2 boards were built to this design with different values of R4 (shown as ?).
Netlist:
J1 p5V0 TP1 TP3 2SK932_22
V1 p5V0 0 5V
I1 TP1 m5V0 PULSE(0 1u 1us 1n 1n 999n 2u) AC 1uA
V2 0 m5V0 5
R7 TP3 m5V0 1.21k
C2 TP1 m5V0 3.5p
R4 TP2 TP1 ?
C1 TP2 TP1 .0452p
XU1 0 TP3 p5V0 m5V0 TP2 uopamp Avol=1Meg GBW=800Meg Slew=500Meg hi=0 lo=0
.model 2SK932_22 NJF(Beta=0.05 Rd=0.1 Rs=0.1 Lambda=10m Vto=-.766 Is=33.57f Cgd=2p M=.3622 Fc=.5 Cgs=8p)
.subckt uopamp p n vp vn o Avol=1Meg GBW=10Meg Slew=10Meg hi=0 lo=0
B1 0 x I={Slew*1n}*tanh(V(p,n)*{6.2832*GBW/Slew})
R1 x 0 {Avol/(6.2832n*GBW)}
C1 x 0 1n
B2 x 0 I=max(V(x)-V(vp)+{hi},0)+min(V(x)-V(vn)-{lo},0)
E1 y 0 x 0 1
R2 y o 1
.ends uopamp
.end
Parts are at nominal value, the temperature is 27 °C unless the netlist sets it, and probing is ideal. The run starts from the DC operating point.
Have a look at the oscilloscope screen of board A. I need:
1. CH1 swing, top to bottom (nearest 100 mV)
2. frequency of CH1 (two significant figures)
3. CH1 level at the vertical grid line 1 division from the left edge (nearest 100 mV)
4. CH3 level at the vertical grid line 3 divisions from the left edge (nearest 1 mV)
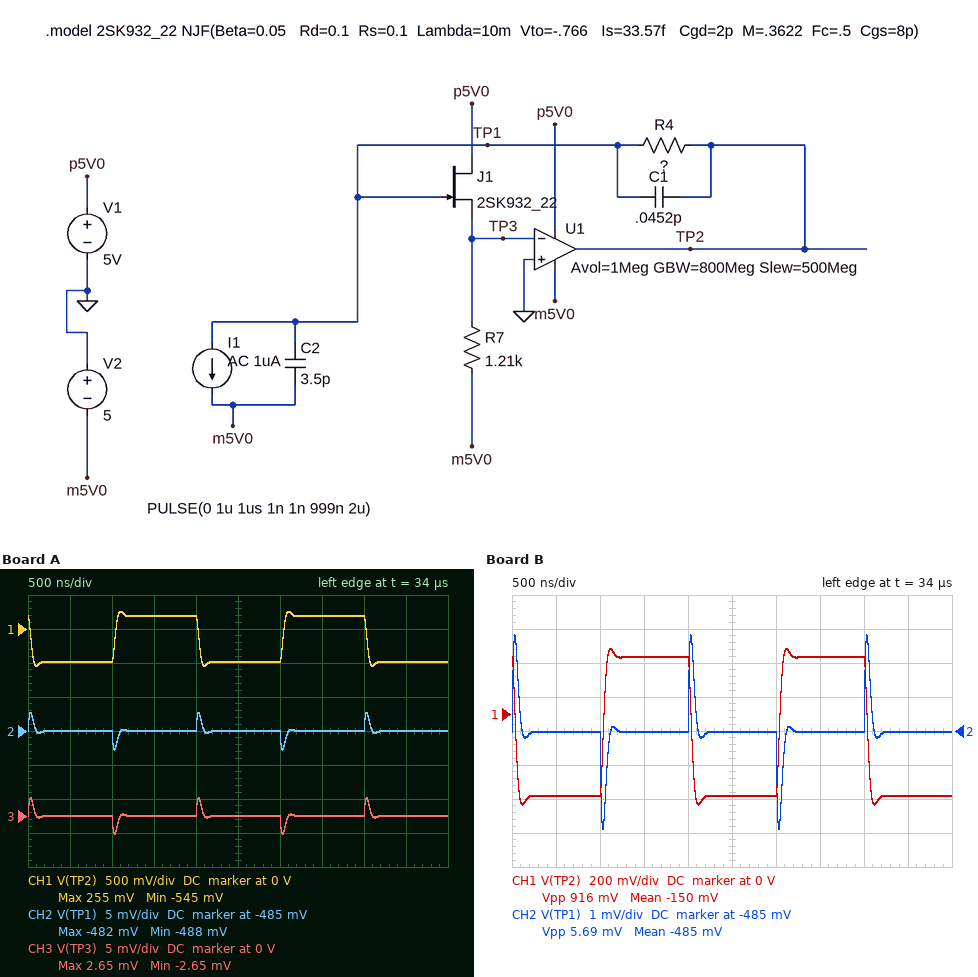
800 mV
500 kHz
-500 mV
0 V
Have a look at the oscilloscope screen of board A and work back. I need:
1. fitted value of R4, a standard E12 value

680 kΩ
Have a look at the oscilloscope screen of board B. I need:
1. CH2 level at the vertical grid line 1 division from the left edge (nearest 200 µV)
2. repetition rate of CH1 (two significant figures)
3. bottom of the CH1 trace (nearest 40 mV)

-485.0 mV
500 kHz
-520 mV
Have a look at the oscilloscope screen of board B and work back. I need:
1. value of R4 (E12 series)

820 kΩ
